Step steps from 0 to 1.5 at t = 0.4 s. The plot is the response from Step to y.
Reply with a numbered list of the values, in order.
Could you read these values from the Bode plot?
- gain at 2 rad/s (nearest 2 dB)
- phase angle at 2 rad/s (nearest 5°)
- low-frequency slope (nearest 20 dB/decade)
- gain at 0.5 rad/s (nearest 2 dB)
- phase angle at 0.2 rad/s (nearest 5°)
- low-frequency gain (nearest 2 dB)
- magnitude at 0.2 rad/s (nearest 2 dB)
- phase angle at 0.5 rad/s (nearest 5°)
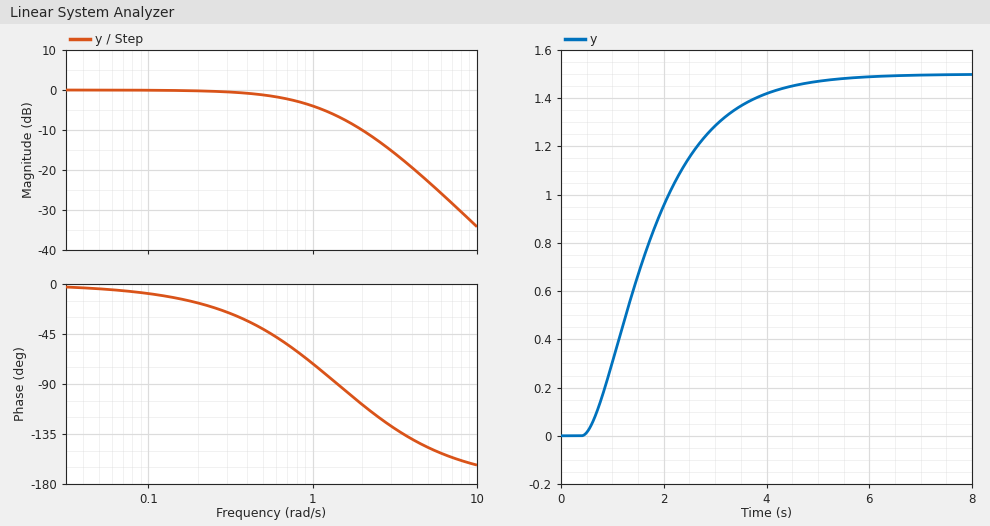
1. -10 dB
2. -110°
3. 0 dB/decade
4. -2 dB
5. -15°
6. 0 dB
7. 0 dB
8. -40°
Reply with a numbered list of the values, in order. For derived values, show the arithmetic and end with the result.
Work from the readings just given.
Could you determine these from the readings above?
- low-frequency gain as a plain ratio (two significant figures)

1. 10^(0 / 20) = 1.0
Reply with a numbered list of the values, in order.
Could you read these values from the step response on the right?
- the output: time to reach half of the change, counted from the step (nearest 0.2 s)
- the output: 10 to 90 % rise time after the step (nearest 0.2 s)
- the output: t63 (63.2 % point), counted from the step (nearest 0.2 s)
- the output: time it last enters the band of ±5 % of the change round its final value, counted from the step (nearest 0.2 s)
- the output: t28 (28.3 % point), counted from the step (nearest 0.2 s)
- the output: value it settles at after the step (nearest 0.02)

1. 1.2 s
2. 2.6 s
3. 1.6 s
4. 3.6 s
5. 0.8 s
6. 1.50
